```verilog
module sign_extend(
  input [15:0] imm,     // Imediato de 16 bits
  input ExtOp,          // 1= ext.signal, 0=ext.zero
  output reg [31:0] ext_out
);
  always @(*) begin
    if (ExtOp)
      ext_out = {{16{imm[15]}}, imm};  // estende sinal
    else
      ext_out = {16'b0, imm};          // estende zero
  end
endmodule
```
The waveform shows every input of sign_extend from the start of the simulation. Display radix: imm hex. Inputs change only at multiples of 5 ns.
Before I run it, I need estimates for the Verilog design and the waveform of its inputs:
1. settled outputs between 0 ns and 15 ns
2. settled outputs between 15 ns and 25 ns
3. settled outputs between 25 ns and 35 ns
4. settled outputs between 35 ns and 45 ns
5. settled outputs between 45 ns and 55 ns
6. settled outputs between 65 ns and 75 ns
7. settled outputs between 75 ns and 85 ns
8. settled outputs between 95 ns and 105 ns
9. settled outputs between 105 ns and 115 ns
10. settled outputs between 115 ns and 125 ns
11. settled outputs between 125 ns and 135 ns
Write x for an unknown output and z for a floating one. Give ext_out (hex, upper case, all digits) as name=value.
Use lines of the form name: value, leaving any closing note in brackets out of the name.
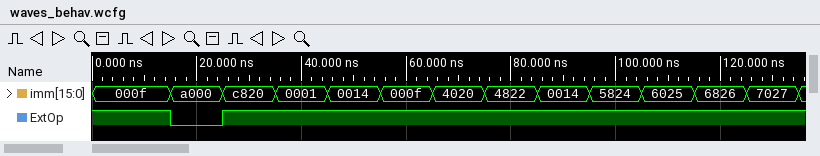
settled outputs between 0 ns and 15 ns: ext_out=0000000F
settled outputs between 15 ns and 25 ns: ext_out=0000A000
settled outputs between 25 ns and 35 ns: ext_out=FFFFC820
settled outputs between 35 ns and 45 ns: ext_out=00000001
settled outputs between 45 ns and 55 ns: ext_out=00000014
settled outputs between 65 ns and 75 ns: ext_out=00004020
settled outputs between 75 ns and 85 ns: ext_out=00004822
settled outputs between 95 ns and 105 ns: ext_out=00005824
settled outputs between 105 ns and 115 ns: ext_out=00006025
settled outputs between 115 ns and 125 ns: ext_out=00006826
settled outputs between 125 ns and 135 ns: ext_out=00007027
